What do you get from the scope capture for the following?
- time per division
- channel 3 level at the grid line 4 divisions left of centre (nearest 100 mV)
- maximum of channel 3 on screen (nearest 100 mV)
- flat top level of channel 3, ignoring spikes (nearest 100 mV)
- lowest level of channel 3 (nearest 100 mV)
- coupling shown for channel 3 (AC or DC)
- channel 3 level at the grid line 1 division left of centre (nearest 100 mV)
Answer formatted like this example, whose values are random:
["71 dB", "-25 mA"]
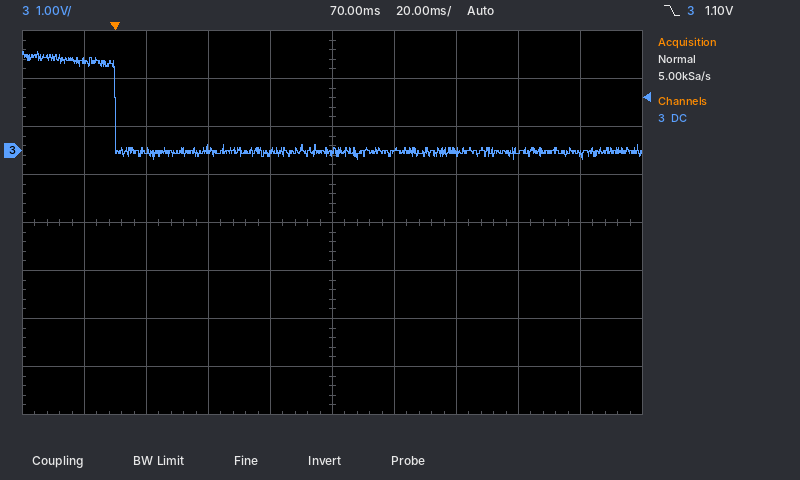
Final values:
["20 ms", "1.9 V", "2.1 V", "1.9 V", "-200 mV", "DC", "0.0 V"]
